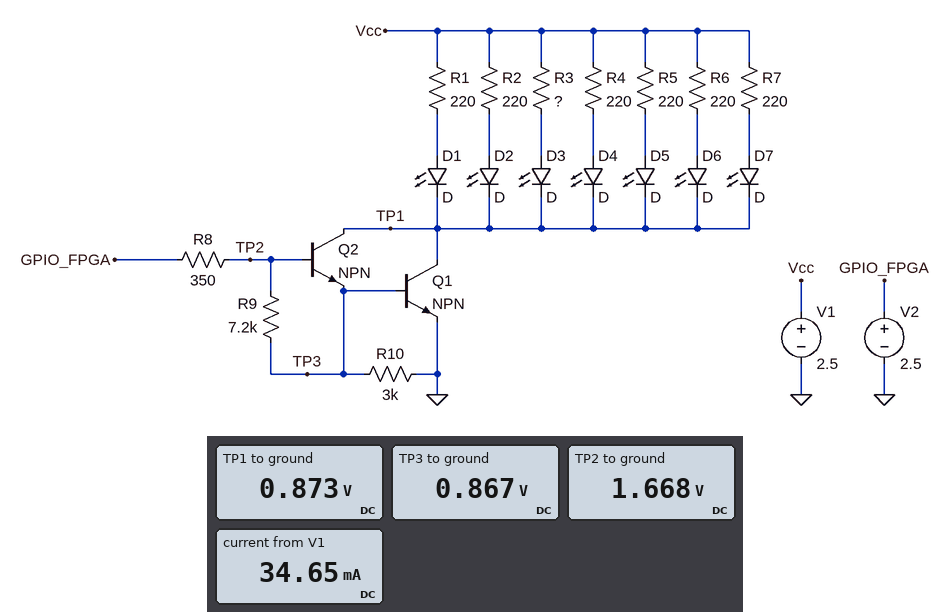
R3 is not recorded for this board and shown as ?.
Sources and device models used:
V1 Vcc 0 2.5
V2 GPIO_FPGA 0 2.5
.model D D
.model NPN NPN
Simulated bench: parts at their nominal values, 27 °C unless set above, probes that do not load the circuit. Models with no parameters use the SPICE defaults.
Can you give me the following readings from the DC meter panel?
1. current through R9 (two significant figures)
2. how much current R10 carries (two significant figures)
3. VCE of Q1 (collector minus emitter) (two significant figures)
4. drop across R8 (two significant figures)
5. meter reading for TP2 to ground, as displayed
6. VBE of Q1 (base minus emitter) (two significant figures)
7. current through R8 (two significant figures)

110 µA
290 µA
870 mV
830 mV
1.668 V
870 mV
2.4 mA
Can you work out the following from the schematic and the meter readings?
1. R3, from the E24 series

100 Ω
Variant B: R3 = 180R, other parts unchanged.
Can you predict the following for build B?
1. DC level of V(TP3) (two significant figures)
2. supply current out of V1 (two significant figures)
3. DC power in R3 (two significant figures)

860 mV
31 mA
4.8 mW
